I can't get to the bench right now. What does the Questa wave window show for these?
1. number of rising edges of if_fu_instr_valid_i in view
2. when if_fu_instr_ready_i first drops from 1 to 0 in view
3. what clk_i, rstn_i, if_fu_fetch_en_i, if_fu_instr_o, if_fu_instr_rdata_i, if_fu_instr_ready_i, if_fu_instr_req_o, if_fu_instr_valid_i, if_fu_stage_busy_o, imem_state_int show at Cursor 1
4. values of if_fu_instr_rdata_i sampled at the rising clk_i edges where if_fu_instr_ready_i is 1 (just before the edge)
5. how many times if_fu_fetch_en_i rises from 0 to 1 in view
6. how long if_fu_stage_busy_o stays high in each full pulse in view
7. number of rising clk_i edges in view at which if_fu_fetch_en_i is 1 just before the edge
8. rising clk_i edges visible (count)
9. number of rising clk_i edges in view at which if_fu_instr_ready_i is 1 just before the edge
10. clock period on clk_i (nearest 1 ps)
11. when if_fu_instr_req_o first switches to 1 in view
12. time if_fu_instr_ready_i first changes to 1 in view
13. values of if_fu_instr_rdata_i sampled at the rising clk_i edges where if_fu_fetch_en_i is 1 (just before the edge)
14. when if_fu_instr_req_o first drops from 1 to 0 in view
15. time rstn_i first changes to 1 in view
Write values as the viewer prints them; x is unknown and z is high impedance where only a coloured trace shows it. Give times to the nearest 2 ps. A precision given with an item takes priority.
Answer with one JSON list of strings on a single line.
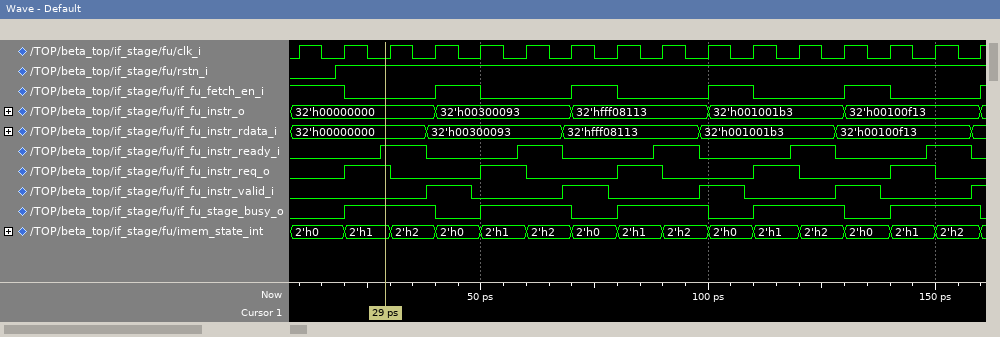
["5", "38 ps", "clk_i=0, rstn_i=1, if_fu_fetch_en_i=0, if_fu_instr_o=32'h00000000, if_fu_instr_rdata_i=32'h00000000, if_fu_instr_ready_i=1, if_fu_instr_req_o=1, if_fu_instr_valid_i=0, if_fu_stage_busy_o=1, imem_state_int=2'h1", "32'h00000000, 32'h00300093, 32'hfff08113, 32'h001001b3, 32'h00100f13", "5", "20 ps, 20 ps, 20 ps, 20 ps, 20 ps", "6", "16", "5", "10 ps", "20 ps", "28 ps", "32'h00000000, 32'h00000000, 32'h00300093, 32'hfff08113, 32'h001001b3, 32'h00100f13", "30 ps", "18 ps"]
